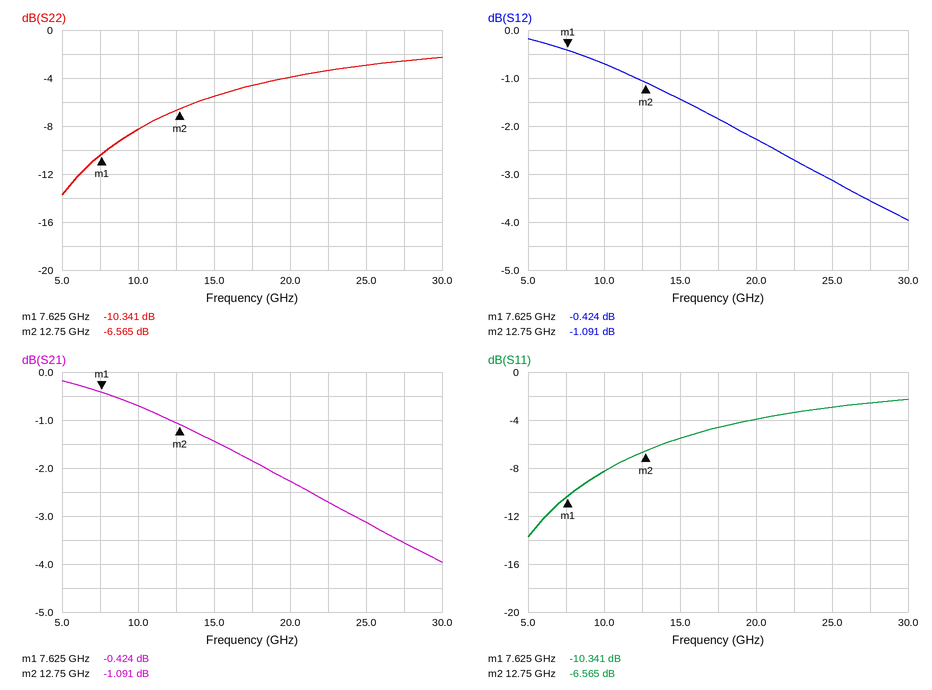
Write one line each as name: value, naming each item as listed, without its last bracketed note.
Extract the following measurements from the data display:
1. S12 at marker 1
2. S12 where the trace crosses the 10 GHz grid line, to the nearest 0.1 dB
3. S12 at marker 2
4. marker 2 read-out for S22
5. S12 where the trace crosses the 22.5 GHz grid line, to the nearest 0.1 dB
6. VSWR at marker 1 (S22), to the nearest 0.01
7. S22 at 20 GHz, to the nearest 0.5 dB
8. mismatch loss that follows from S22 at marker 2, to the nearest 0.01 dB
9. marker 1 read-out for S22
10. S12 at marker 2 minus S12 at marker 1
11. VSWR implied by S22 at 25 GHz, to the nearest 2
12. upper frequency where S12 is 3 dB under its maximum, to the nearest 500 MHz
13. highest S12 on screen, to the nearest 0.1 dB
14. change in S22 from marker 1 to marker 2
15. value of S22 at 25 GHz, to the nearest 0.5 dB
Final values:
S12 at marker 1: -0.424 dB
S12 where the trace crosses the 10 GHz grid line, to the nearest 0.1 dB: -0.7 dB
S12 at marker 2: -1.091 dB
marker 2 read-out for S22: -6.565 dB
S12 where the trace crosses the 22.5 GHz grid line, to the nearest 0.1 dB: -2.7 dB
VSWR at marker 1 (S22), to the nearest 0.01: 1.87
S22 at 20 GHz, to the nearest 0.5 dB: -4.0 dB
mismatch loss that follows from S22 at marker 2, to the nearest 0.01 dB: 1.08 dB
marker 1 read-out for S22: -10.341 dB
S12 at marker 2 minus S12 at marker 1: -0.667 dB
VSWR implied by S22 at 25 GHz, to the nearest 2: 6
upper frequency where S12 is 3 dB under its maximum, to the nearest 500 MHz: 25.5 GHz
highest S12 on screen, to the nearest 0.1 dB: -0.2 dB
change in S22 from marker 1 to marker 2: 3.776 dB
value of S22 at 25 GHz, to the nearest 0.5 dB: -3.0 dB
